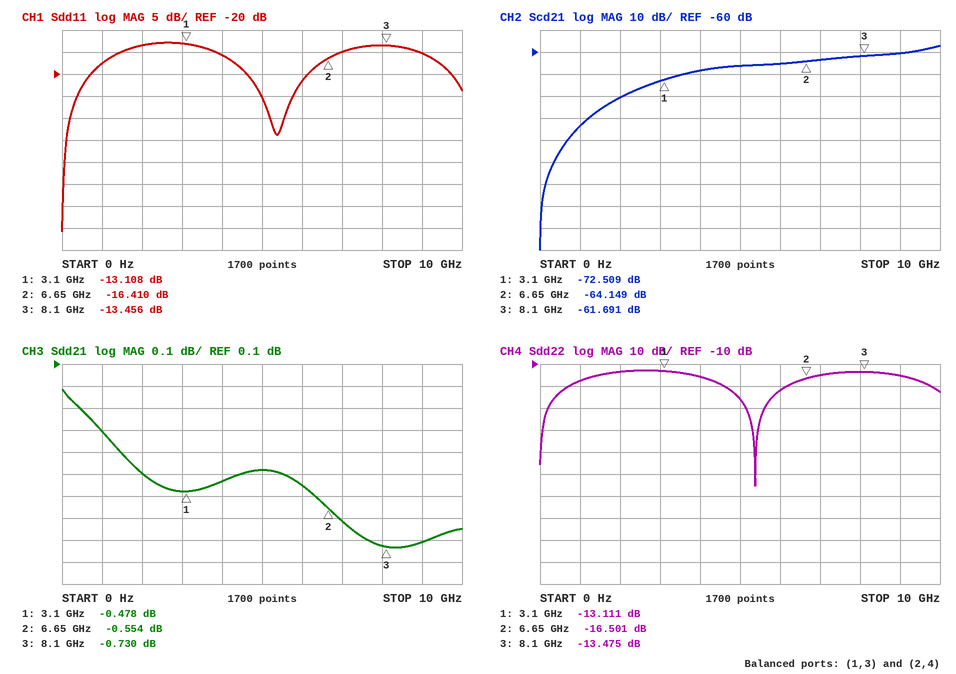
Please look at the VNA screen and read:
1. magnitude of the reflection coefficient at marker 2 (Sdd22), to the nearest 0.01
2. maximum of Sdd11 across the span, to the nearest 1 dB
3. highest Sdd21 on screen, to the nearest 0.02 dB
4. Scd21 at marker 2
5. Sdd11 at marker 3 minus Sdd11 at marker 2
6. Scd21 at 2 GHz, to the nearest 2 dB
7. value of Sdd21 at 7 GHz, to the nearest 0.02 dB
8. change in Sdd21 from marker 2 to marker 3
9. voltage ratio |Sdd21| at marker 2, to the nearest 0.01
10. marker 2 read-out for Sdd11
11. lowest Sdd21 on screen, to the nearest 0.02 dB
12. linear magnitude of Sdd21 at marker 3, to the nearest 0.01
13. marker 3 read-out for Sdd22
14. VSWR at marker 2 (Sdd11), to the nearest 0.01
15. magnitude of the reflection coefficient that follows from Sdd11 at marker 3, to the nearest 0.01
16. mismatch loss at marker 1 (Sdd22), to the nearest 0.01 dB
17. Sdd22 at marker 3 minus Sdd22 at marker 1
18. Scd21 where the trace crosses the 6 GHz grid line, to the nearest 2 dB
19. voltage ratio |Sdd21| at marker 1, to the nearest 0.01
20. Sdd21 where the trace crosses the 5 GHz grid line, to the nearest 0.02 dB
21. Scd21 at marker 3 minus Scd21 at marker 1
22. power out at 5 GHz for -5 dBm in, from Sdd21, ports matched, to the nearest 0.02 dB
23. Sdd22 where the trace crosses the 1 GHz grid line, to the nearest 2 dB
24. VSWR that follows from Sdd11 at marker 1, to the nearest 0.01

0.15
-13 dB
-0.02 dB
-64.149 dB
2.954 dB
-80 dB
-0.62 dB
-0.176 dB
0.94
-16.410 dB
-0.74 dB
0.92
-13.475 dB
1.36
0.21
0.22 dB
-0.364 dB
-66 dB
0.95
-0.38 dB
10.818 dB
-5.38 dBm
-18 dB
1.57
